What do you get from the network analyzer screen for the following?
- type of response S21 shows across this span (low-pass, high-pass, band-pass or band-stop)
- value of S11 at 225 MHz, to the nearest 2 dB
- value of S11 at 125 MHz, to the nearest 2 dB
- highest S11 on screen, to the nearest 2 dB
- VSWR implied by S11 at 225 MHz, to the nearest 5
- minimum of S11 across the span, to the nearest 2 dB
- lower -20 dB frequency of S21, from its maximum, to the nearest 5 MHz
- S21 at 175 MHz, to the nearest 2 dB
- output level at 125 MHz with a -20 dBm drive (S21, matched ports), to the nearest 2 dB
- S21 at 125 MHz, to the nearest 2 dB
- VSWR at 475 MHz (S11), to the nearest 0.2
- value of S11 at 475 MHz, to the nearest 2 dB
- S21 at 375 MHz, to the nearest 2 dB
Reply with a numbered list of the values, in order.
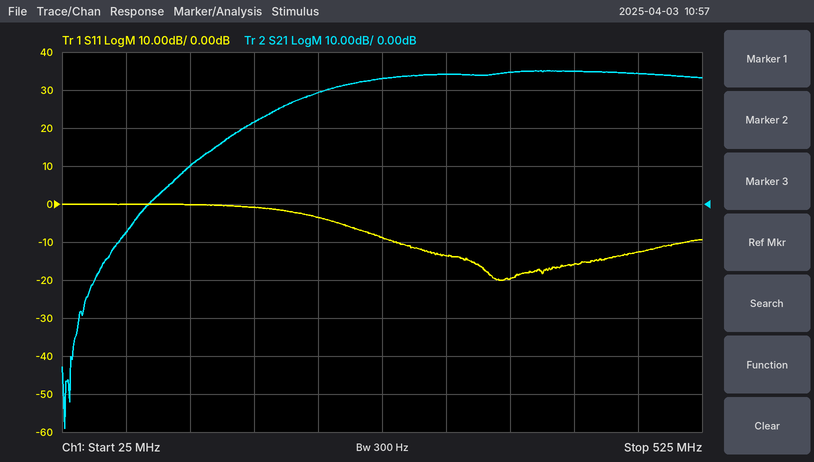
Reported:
1. high-pass
2. -4 dB
3. 0 dB
4. 0 dB
5. 5
6. -20 dB
7. 145 MHz
8. 22 dB
9. -10 dBm
10. 10 dB
11. 1.6
12. -12 dB
13. 34 dB
